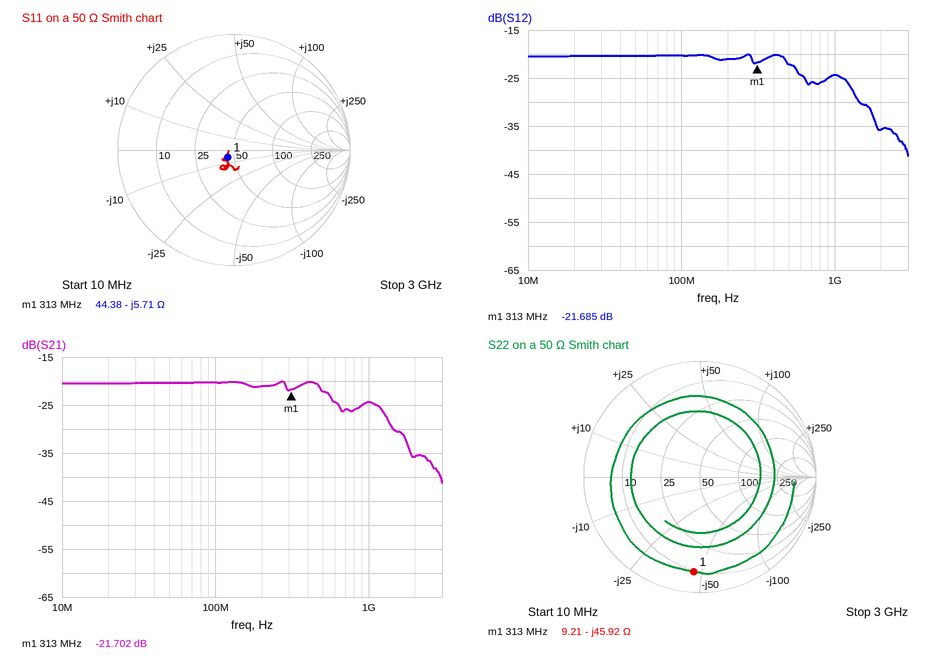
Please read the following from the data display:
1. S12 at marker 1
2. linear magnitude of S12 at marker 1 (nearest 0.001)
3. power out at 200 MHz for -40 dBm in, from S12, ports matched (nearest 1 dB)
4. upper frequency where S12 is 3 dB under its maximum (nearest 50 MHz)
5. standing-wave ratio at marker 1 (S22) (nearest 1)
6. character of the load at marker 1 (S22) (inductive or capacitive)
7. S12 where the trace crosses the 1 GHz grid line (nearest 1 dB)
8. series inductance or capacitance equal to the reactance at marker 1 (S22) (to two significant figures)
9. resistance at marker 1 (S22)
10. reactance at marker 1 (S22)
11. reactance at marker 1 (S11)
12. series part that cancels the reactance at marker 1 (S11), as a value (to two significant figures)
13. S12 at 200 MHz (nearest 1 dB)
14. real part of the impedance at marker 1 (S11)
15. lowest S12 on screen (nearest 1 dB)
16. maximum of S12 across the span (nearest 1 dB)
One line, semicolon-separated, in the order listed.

-21.685 dB; 0.082; -61 dBm; 550 MHz; 10; capacitive; -24 dB; 11 pF; 9.21 Ω; -45.92 Ω; -5.71 Ω; 2.9 nH; -21 dB; 44.38 Ω; -41 dB; -20 dB
